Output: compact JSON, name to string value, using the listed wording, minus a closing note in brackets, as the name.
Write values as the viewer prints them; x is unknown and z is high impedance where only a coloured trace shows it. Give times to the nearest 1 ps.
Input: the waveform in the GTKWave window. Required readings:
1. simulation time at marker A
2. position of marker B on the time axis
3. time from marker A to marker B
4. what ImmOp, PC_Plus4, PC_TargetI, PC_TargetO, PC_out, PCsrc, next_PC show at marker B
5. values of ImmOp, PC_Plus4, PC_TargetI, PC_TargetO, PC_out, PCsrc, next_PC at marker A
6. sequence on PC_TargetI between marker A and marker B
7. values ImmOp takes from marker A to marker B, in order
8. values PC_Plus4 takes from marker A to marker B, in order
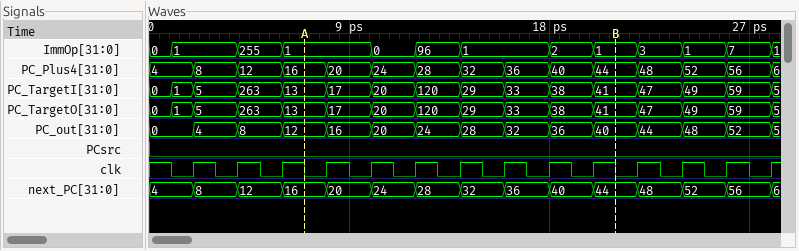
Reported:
{"simulation time at marker A": "7 ps", "position of marker B on the time axis": "21 ps", "time from marker A to marker B": "14 ps", "what ImmOp, PC_Plus4, PC_TargetI, PC_TargetO, PC_out, PCsrc, next_PC show at marker B": "ImmOp=1, PC_Plus4=44, PC_TargetI=41, PC_TargetO=41, PC_out=40, PCsrc=0, next_PC=44", "values of ImmOp, PC_Plus4, PC_TargetI, PC_TargetO, PC_out, PCsrc, next_PC at marker A": "ImmOp=1, PC_Plus4=16, PC_TargetI=13, PC_TargetO=13, PC_out=12, PCsrc=0, next_PC=16", "sequence on PC_TargetI between marker A and marker B": "13, 17, 20, 120, 29, 33, 38, 41", "values ImmOp takes from marker A to marker B, in order": "1, 0, 96, 1, 2, 1", "values PC_Plus4 takes from marker A to marker B, in order": "16, 20, 24, 28, 32, 36, 40, 44"}
